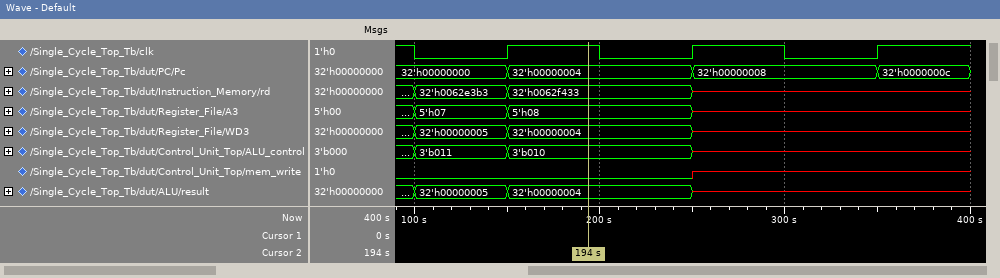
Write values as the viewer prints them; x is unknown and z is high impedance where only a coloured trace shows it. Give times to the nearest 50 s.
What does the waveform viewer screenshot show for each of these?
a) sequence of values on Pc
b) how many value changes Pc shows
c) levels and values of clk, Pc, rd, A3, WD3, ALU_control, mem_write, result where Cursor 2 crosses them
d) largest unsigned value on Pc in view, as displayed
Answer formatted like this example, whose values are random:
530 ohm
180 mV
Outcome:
32'h00000000, 32'h00000004, 32'h00000008, 32'h0000000c
3
clk=1, Pc=32'h00000004, rd=32'h0062f433, A3=5'h08, WD3=32'h00000004, ALU_control=3'b010, mem_write=0, result=32'h00000004
32'h0000000c
